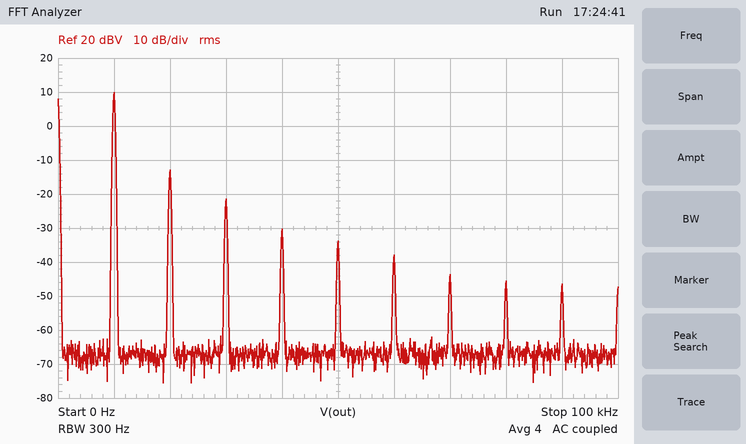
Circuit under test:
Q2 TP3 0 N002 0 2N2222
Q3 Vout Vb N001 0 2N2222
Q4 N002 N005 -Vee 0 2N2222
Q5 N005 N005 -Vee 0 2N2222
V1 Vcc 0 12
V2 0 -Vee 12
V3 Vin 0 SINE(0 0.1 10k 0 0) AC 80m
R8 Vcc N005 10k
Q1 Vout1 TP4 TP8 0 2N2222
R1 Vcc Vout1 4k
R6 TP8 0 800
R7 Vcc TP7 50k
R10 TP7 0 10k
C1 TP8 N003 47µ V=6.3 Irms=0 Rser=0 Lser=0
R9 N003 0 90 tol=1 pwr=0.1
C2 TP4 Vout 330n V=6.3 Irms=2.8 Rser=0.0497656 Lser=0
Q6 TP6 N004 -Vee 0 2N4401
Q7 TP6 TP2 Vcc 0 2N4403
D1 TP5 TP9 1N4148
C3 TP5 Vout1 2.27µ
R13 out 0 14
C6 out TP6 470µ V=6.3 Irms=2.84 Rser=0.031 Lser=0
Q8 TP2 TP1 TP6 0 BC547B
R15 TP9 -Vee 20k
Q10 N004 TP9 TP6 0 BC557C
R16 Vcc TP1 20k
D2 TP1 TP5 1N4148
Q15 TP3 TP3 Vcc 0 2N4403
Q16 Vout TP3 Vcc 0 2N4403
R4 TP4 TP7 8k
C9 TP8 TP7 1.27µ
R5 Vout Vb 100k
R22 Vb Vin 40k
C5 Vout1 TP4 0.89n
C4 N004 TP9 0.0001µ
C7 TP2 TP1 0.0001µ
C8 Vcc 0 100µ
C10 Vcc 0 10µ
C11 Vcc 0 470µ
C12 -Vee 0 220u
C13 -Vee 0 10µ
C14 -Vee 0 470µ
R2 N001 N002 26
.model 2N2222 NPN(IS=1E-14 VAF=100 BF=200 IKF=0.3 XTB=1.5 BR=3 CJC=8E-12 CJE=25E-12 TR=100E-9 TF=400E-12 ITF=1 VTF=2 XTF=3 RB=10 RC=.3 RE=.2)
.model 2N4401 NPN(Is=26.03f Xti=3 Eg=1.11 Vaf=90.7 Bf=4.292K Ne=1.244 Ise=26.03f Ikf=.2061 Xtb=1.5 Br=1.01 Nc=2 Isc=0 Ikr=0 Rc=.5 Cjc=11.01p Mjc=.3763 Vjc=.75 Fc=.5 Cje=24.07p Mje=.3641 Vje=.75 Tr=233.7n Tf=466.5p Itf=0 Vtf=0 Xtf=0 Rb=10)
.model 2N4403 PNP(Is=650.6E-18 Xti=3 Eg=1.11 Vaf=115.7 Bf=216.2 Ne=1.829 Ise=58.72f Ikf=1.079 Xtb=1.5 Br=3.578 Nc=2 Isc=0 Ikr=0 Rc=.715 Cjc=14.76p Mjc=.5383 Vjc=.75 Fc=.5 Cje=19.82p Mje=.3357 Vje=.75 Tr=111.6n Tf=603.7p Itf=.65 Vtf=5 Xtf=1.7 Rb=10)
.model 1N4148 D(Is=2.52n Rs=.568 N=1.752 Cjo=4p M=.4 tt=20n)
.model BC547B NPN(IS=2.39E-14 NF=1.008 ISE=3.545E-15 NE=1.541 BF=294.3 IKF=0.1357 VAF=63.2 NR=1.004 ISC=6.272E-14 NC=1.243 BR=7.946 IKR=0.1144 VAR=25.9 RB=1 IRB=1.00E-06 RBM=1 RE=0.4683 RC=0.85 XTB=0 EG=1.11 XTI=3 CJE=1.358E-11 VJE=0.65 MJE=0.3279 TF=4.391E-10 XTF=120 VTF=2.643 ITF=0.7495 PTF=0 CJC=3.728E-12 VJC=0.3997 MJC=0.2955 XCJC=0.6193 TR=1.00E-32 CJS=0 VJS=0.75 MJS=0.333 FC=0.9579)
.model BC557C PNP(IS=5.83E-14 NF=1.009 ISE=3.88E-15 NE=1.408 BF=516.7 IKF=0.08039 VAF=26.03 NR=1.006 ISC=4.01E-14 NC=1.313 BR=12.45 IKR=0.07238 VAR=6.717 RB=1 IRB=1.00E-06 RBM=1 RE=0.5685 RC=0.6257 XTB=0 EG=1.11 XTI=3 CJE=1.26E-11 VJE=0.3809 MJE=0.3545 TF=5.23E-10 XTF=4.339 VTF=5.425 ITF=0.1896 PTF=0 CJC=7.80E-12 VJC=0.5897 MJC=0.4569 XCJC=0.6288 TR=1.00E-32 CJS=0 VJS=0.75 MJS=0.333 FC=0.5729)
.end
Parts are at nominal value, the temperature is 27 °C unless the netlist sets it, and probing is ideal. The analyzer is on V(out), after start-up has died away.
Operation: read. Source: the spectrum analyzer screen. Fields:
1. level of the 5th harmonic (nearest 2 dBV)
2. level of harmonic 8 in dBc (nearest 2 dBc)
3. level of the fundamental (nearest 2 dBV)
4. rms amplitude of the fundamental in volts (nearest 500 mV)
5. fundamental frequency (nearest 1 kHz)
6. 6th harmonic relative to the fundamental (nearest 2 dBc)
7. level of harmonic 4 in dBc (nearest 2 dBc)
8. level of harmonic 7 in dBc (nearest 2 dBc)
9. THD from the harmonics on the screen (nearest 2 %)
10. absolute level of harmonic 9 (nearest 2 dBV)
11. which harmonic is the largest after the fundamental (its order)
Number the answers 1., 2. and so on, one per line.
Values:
1. -34 dBV
2. -56 dBc
3. 10 dBV
4. 3.0 V
5. 10 kHz
6. -48 dBc
7. -40 dBc
8. -54 dBc
9. 8 %
10. -46 dBV
11. 2
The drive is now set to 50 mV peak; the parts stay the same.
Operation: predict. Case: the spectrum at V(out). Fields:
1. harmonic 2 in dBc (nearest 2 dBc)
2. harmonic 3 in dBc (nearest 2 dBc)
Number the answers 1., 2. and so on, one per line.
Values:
1. -36 dBc
2. -56 dBc
